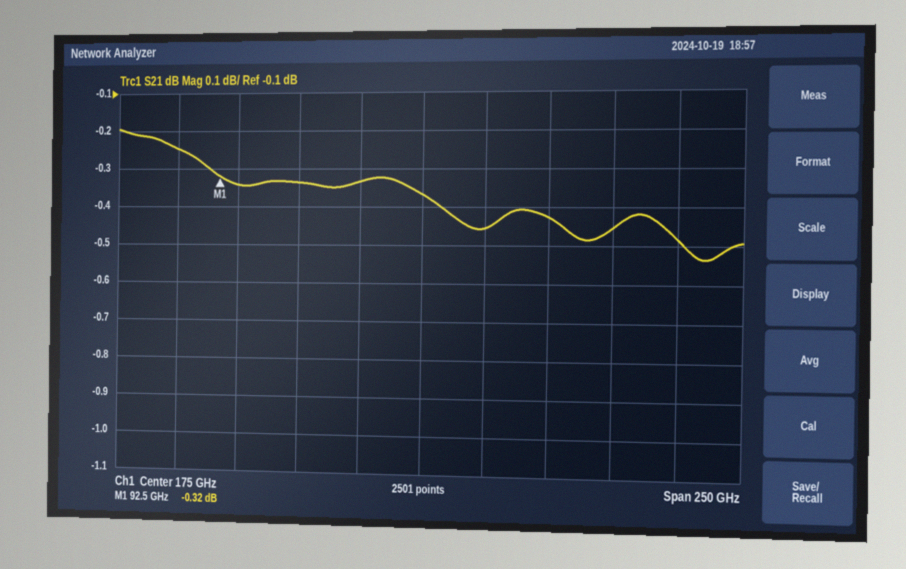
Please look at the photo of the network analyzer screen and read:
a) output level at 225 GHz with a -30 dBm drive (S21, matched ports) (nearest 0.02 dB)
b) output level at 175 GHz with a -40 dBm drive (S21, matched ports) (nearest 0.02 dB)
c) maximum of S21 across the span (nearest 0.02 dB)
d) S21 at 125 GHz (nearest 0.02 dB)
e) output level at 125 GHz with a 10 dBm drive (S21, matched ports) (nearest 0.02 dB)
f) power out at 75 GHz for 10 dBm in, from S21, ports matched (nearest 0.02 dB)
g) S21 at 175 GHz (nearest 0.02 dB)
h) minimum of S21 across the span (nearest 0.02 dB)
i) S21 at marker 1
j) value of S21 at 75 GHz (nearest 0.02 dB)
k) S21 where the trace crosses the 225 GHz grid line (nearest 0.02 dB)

-30.42 dBm
-40.36 dBm
-0.20 dB
-0.34 dB
9.66 dBm
9.76 dBm
-0.36 dB
-0.54 dB
-0.32 dB
-0.24 dB
-0.42 dB
